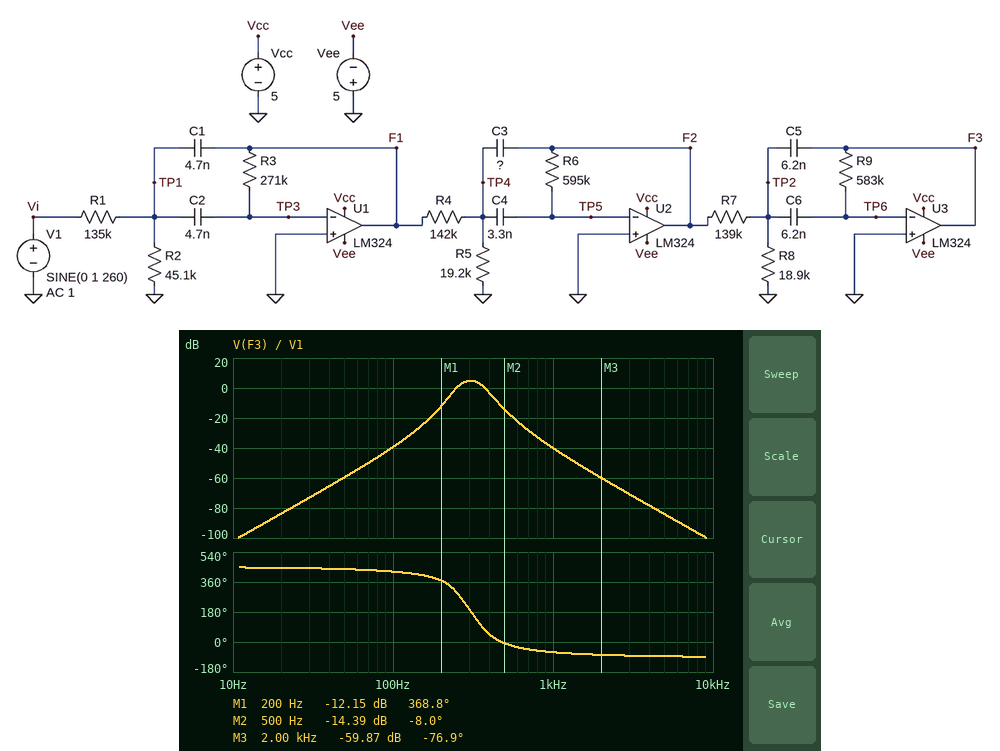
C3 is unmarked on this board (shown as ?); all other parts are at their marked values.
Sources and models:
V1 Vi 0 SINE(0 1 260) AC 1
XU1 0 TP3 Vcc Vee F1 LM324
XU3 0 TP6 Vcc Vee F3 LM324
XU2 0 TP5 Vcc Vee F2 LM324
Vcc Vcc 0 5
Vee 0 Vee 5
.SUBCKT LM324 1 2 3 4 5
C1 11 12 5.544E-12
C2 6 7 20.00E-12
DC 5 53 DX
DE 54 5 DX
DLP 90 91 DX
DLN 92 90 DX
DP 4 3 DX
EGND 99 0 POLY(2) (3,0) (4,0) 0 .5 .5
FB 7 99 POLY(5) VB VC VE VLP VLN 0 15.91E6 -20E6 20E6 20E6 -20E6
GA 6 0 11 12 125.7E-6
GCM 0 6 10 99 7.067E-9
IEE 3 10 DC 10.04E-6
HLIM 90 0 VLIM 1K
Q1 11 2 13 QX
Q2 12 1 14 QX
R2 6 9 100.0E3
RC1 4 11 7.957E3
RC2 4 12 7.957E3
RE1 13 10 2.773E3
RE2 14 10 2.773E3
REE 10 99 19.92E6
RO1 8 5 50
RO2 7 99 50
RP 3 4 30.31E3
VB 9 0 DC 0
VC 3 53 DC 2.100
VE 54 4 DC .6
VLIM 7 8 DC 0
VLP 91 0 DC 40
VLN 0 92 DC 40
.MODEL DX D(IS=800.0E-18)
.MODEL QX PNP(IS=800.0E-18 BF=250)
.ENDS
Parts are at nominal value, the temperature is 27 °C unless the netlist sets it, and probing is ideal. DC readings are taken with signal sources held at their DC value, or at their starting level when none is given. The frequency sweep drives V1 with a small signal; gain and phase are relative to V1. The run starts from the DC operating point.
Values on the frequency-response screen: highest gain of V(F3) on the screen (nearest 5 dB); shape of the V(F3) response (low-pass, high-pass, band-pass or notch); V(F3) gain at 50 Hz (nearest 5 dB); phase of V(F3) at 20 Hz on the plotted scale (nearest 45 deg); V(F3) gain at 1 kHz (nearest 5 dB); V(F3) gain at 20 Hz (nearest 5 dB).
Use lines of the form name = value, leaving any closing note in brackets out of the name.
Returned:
highest gain of V(F3) on the screen = 5 dB
shape of the V(F3) response = band-pass
V(F3) gain at 50 Hz = -60 dB
phase of V(F3) at 20 Hz on the plotted scale = 450 deg
V(F3) gain at 1 kHz = -40 dB
V(F3) gain at 20 Hz = -85 dB
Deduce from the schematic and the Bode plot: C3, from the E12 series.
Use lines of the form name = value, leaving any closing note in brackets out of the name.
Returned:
C3, from the E12 series = 6.8 nF
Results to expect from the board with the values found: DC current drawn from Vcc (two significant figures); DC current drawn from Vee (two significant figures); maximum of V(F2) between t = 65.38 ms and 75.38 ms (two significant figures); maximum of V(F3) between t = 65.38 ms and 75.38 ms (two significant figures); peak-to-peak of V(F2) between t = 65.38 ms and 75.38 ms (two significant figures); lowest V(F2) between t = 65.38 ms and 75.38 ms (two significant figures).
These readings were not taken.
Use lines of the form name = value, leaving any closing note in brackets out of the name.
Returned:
DC current drawn from Vcc = 1.0 mA
DC current drawn from Vee = 1.0 mA
maximum of V(F2) between t = 65.38 ms and 75.38 ms = 580 mV
maximum of V(F3) between t = 65.38 ms and 75.38 ms = 1.2 V
peak-to-peak of V(F2) between t = 65.38 ms and 75.38 ms = 1.2 V
lowest V(F2) between t = 65.38 ms and 75.38 ms = -600 mV
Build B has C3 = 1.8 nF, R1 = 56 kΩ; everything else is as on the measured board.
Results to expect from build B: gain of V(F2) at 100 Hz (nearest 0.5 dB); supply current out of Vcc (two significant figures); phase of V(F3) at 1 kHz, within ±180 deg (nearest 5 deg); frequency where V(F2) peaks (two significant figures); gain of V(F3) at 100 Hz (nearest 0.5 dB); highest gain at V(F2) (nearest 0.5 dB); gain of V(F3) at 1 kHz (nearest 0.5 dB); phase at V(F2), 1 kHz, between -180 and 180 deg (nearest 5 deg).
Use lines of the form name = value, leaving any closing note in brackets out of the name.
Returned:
gain of V(F2) at 100 Hz = -25.0 dB
supply current out of Vcc = 1.0 mA
phase of V(F3) at 1 kHz, within ±180 deg = -45 deg
frequency where V(F2) peaks = 610 Hz
gain of V(F3) at 100 Hz = -35.0 dB
highest gain at V(F2) = 11.5 dB
gain of V(F3) at 1 kHz = -17.5 dB
phase at V(F2), 1 kHz, between -180 and 180 deg = -140 deg
